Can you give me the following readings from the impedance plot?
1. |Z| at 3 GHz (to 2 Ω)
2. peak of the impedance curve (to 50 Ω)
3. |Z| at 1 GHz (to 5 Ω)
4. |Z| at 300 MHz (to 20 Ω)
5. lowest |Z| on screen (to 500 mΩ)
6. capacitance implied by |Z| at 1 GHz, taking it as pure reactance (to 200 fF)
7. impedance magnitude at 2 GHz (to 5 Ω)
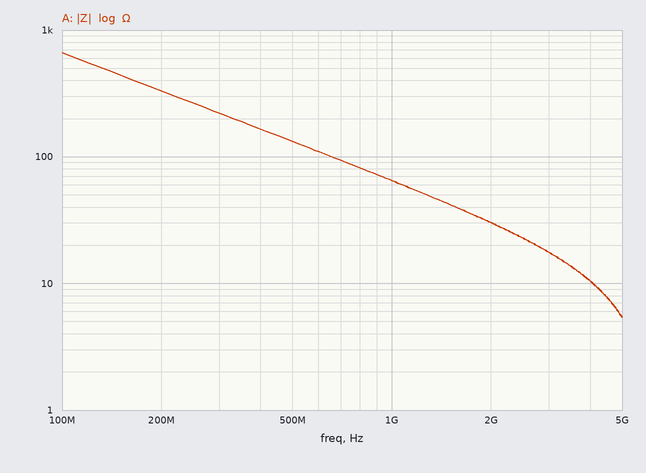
18 Ω
650 Ω
65 Ω
220 Ω
5.5 Ω
2.4 pF
30 Ω
